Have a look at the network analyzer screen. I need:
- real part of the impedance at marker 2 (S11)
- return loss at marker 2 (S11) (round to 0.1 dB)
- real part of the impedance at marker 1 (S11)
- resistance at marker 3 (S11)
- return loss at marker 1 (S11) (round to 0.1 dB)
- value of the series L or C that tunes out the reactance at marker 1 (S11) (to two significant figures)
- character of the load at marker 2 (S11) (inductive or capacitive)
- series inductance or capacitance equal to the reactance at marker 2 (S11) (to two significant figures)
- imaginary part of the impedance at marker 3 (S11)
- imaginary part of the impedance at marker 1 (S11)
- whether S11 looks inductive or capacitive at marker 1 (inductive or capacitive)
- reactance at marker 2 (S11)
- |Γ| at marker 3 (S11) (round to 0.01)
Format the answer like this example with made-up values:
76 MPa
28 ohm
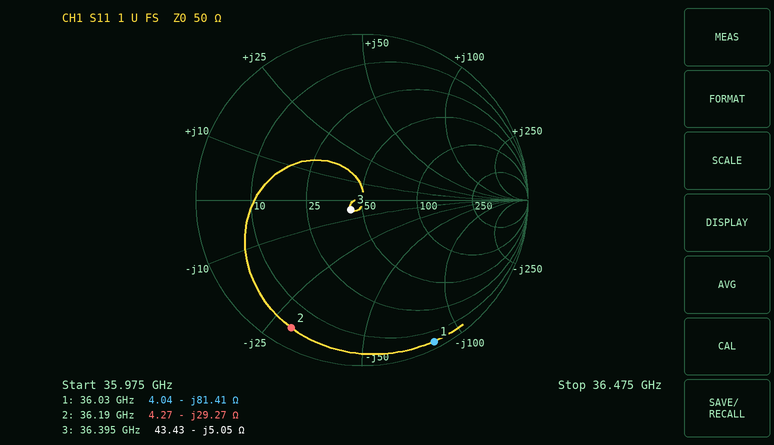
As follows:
4.27 Ω
1.1 dB
4.04 Ω
43.43 Ω
0.4 dB
360 pH
capacitive
150 fF
-5.05 Ω
-81.41 Ω
capacitive
-29.27 Ω
0.09
